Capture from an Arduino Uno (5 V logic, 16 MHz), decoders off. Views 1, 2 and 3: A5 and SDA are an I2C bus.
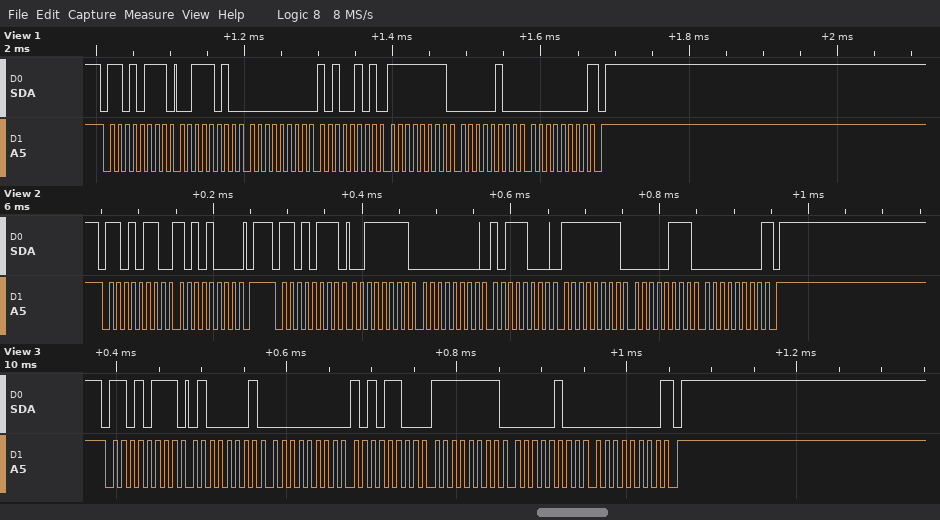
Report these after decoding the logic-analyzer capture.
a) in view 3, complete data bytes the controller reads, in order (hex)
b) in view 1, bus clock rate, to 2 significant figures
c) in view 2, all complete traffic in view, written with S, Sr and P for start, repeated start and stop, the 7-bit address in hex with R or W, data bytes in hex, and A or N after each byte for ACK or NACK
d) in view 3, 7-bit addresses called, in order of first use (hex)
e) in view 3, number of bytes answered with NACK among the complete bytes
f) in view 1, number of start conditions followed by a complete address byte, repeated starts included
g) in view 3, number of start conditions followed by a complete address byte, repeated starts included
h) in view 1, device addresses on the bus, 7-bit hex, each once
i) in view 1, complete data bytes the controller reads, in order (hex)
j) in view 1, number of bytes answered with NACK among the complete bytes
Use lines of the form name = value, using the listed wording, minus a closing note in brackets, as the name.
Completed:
in view 3, complete data bytes the controller reads, in order = 41 00 AC FF 04 00
in view 1, bus clock rate, to 2 significant figures = 100 kHz
in view 2, all complete traffic in view, written with S, Sr and P for start, repeated start and stop, the 7-bit address in hex with R or W, data bytes in hex, and A or N after each byte for ACK or NACK = S 6BW A A8 A P S 6BR A 3F A 00 A B8 A FF A 07 A 00 N P
in view 3, 7-bit addresses called, in order of first use = 0x6B
in view 3, number of bytes answered with NACK among the complete bytes = 1
in view 1, number of start conditions followed by a complete address byte, repeated starts included = 1
in view 3, number of start conditions followed by a complete address byte, repeated starts included = 1
in view 1, device addresses on the bus, 7-bit hex, each once = 0x6B
in view 1, complete data bytes the controller reads, in order = 3A 00 A5 FF 04 00
in view 1, number of bytes answered with NACK among the complete bytes = 1
